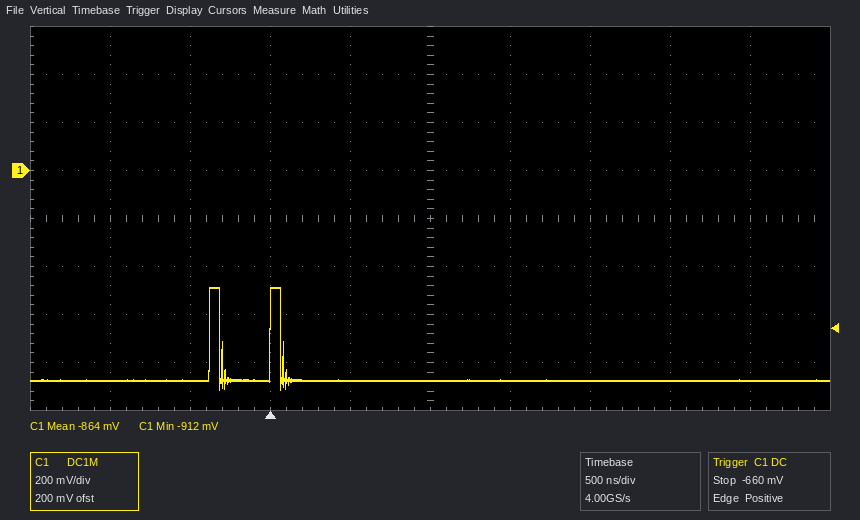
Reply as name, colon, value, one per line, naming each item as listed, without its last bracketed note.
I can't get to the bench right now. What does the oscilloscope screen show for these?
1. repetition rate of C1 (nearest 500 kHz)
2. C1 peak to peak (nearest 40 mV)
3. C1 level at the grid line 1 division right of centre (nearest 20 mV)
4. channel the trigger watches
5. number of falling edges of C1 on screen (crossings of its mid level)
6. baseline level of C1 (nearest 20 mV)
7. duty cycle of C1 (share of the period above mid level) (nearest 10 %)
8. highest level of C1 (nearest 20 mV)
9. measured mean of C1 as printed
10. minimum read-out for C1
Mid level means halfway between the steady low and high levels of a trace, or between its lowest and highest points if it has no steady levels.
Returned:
repetition rate of C1: 2.5 MHz
C1 peak to peak: 440 mV
C1 level at the grid line 1 division right of centre: -880 mV
channel the trigger watches: C1
number of falling edges of C1 on screen: 2
baseline level of C1: -880 mV
duty cycle of C1 (share of the period above mid level): 20 %
highest level of C1: -480 mV
measured mean of C1 as printed: -864 mV
minimum read-out for C1: -912 mV
